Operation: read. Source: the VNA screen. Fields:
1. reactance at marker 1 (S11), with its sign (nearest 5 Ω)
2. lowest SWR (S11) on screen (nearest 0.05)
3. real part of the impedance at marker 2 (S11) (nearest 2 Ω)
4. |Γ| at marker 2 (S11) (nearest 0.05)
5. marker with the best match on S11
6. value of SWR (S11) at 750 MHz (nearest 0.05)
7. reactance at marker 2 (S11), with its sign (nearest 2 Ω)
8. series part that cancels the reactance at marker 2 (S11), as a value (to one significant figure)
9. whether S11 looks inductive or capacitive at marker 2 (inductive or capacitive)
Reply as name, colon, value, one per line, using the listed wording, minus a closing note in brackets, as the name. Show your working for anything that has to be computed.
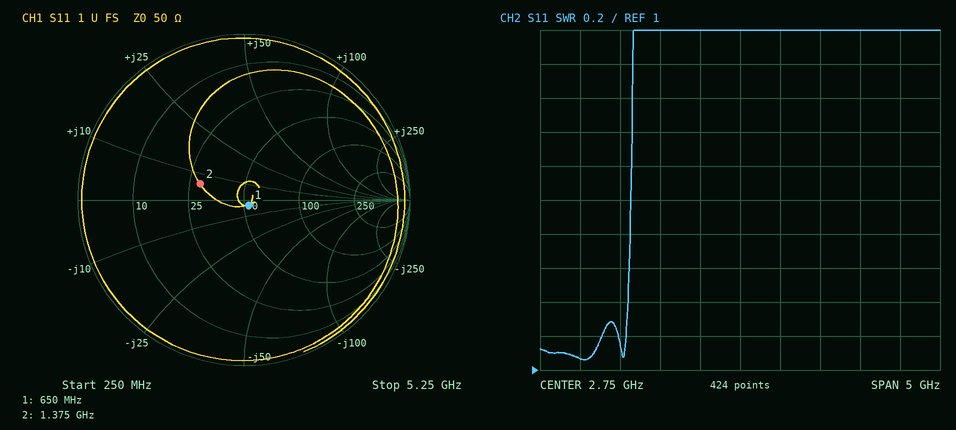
reactance at marker 1 (S11), with its sign: -5 Ω
lowest SWR (S11) on screen: 1.05
real part of the impedance at marker 2 (S11): 28 Ω
|Γ| at marker 2 (S11): 0.30
marker with the best match on S11: marker 1
value of SWR (S11) at 750 MHz: 1.05
reactance at marker 2 (S11), with its sign: +6 Ω
series part that cancels the reactance at marker 2 (S11), as a value: C = 1/(2π × 1.375 GHz × 6 Ω) ≈ 19.3 pF, so 20 pF to one significant figure
whether S11 looks inductive or capacitive at marker 2: inductive
